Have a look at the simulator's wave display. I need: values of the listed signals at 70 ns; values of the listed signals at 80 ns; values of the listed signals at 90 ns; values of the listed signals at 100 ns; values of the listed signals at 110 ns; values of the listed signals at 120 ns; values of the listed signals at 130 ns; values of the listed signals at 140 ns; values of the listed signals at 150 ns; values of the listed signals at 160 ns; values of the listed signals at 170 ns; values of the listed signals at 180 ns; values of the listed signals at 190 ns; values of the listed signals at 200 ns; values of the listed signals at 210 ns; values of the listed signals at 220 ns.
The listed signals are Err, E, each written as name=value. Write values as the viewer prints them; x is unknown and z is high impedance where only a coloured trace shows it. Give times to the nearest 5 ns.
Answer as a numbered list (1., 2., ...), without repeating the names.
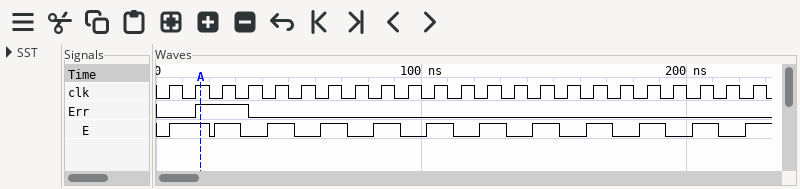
1. Err=0, E=1
2. Err=0, E=0
3. Err=0, E=1
4. Err=0, E=0
5. Err=0, E=1
6. Err=0, E=0
7. Err=0, E=1
8. Err=0, E=0
9. Err=0, E=1
10. Err=0, E=0
11. Err=0, E=1
12. Err=0, E=0
13. Err=0, E=1
14. Err=0, E=0
15. Err=0, E=1
16. Err=0, E=0
